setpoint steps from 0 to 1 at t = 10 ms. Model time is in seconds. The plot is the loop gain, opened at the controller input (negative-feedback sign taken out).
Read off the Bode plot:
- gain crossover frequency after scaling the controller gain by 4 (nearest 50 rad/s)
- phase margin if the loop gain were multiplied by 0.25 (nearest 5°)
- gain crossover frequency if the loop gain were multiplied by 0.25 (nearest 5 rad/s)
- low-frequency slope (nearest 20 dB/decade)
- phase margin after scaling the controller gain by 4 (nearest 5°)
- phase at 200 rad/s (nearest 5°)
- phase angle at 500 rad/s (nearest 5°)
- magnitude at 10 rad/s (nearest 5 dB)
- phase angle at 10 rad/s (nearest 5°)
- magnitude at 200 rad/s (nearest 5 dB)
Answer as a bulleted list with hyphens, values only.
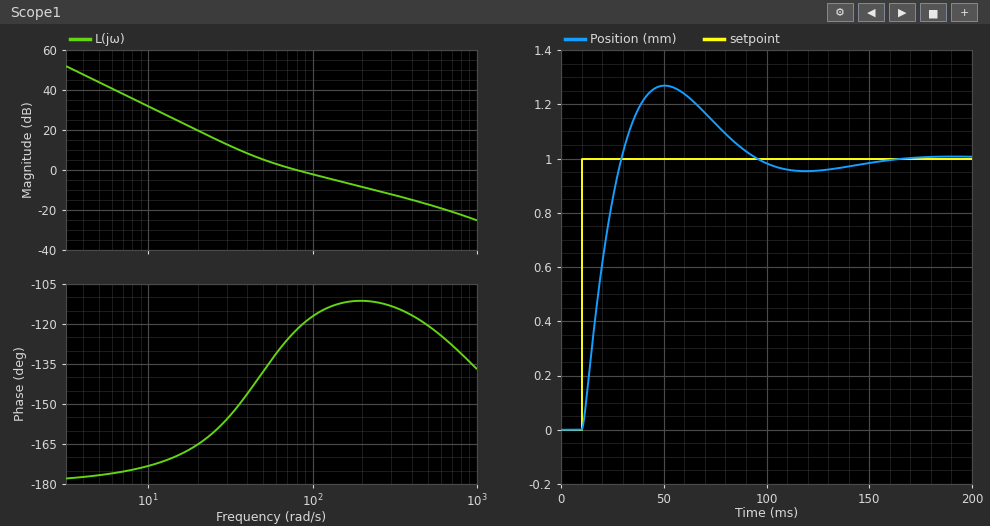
- 300 rad/s
- 25°
- 30 rad/s
- -40 dB/decade
- 65°
- -110°
- -120°
- 30 dB
- -175°
- -10 dB
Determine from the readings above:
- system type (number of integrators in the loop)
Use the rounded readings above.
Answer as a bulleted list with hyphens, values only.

- 2
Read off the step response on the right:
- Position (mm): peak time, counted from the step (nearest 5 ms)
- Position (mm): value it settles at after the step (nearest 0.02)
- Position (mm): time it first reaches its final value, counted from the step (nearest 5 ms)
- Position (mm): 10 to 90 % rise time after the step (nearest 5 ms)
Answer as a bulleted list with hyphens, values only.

- 40 ms
- 1.00
- 20 ms
- 15 ms
